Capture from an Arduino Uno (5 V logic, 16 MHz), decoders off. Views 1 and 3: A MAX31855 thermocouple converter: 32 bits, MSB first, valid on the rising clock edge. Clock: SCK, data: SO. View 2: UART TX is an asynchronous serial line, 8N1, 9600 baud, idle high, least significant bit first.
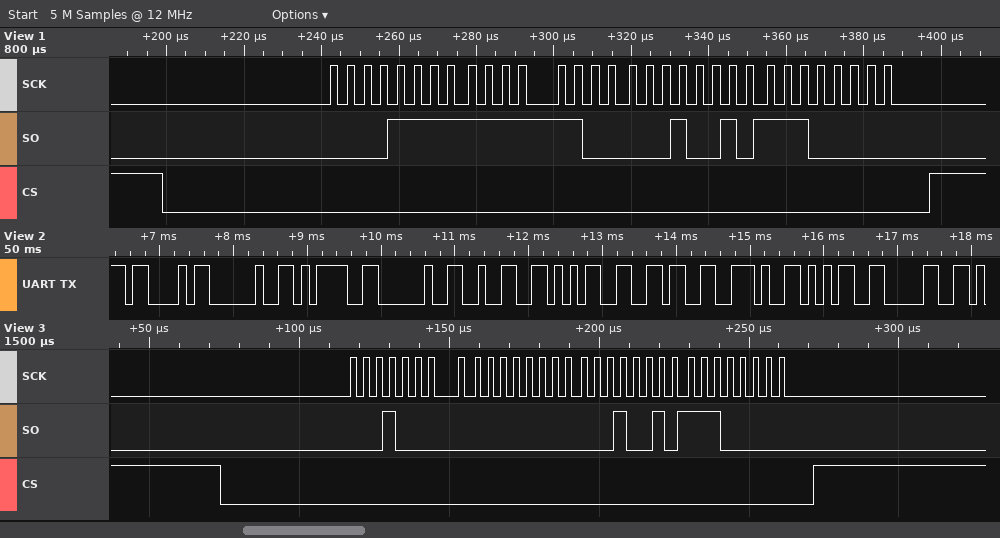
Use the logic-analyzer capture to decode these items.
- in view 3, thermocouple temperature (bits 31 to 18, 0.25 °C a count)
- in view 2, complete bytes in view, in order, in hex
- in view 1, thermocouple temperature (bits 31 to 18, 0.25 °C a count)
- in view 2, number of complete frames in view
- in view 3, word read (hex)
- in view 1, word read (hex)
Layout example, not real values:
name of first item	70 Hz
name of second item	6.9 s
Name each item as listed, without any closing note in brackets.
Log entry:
in view 3, thermocouple temperature	256.00 °C
in view 2, complete bytes in view, in order, in hex	43 20 3D 20 32 35 36 2E 35 30
in view 1, thermocouple temperature	255.75 °C
in view 2, number of complete frames in view	10
in view 3, word read	0x100012E0
in view 1, word read	0x0FFC12E0
